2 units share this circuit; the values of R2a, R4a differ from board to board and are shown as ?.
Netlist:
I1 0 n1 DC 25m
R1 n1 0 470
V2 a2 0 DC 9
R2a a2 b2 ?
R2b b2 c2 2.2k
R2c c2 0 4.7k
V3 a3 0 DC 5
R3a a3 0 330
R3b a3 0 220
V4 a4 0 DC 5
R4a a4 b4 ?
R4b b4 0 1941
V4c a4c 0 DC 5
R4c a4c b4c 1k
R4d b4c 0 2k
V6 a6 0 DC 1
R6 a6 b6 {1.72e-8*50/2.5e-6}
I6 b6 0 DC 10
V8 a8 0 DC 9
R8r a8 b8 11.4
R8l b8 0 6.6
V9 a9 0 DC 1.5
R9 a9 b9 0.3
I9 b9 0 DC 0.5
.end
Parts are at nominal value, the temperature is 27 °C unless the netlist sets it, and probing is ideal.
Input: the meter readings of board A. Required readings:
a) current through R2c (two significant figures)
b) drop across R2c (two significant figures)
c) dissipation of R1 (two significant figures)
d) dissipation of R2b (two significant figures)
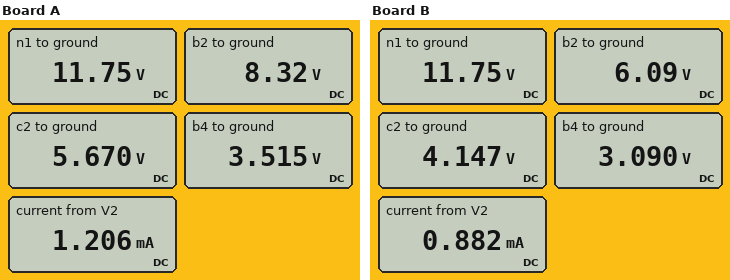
1.2 mA
5.7 V
290 mW
3.2 mW
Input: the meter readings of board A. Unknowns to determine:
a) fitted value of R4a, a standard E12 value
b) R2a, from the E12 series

820 Ω
560 Ω
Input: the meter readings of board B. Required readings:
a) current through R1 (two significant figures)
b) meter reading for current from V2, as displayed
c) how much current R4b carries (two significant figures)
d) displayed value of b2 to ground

25 mA
0.882 mA
1.6 mA
6.09 V
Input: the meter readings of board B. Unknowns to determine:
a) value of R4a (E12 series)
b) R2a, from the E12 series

1.2 kΩ
3.3 kΩ
